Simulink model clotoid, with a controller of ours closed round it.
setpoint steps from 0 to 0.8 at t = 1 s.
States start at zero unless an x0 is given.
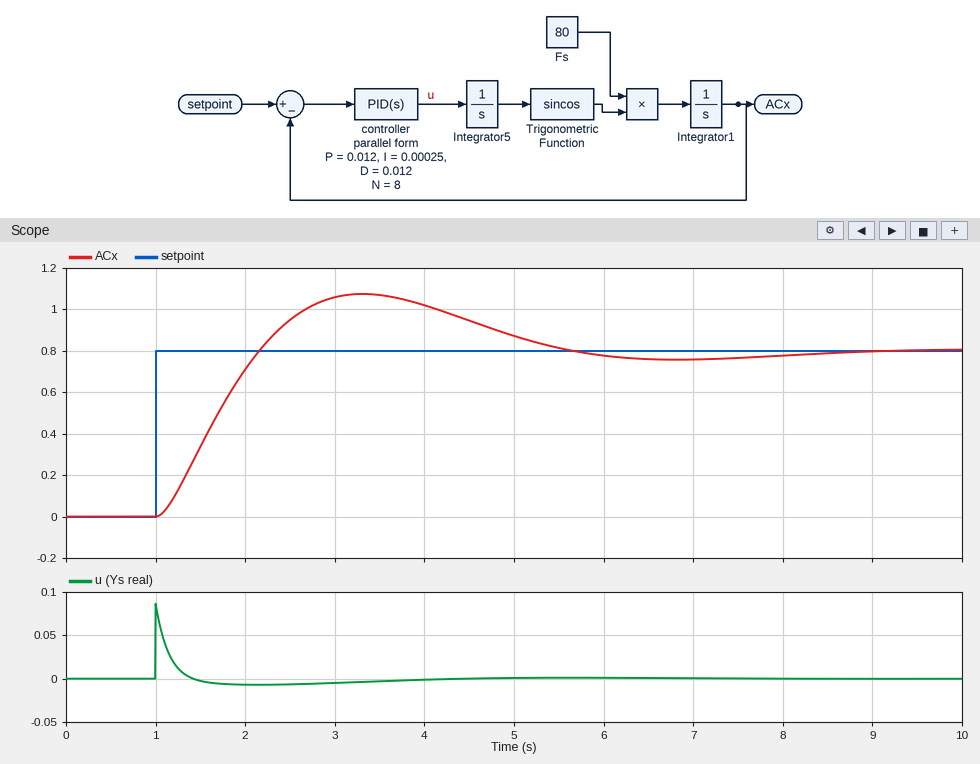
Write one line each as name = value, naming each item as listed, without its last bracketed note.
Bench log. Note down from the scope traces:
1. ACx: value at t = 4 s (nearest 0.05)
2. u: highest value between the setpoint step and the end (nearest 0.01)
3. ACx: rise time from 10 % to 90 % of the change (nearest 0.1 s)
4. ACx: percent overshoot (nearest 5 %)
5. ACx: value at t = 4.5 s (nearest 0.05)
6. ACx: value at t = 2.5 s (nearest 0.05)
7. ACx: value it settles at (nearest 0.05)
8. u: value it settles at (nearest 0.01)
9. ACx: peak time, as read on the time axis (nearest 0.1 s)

ACx: value at t = 4 s = 1.00
u: highest value between the setpoint step and the end = 0.09
ACx: rise time from 10 % to 90 % of the change = 0.8 s
ACx: percent overshoot = 35 %
ACx: value at t = 4.5 s = 0.95
ACx: value at t = 2.5 s = 0.95
ACx: value it settles at = 0.80
u: value it settles at = 0.00
ACx: peak time, as read on the time axis = 3.3 s
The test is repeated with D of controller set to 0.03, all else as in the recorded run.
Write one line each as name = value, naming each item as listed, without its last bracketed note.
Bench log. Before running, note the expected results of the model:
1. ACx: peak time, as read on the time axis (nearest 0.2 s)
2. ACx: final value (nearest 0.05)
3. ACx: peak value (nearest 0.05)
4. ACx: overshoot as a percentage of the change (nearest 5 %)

ACx: peak time, as read on the time axis = 2.4 s
ACx: final value = 0.80
ACx: peak value = 0.90
ACx: overshoot as a percentage of the change = 15 %
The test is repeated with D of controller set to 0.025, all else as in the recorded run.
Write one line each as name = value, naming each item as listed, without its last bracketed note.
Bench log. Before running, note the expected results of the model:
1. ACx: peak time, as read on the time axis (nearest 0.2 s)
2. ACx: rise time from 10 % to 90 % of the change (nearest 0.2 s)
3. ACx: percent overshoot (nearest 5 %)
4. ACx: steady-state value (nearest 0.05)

ACx: peak time, as read on the time axis = 2.6 s
ACx: rise time from 10 % to 90 % of the change = 0.6 s
ACx: percent overshoot = 15 %
ACx: steady-state value = 0.80
